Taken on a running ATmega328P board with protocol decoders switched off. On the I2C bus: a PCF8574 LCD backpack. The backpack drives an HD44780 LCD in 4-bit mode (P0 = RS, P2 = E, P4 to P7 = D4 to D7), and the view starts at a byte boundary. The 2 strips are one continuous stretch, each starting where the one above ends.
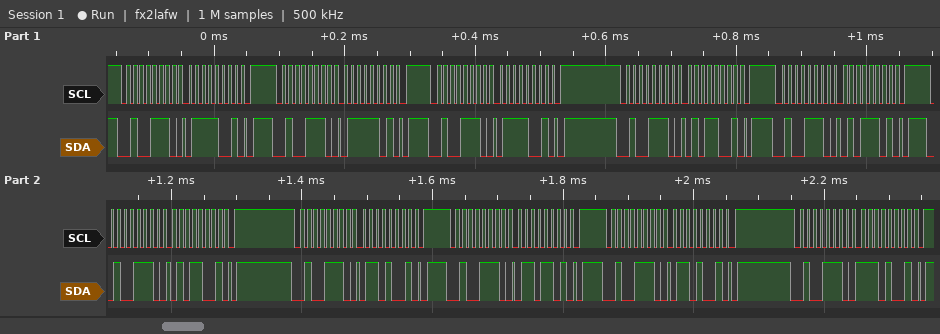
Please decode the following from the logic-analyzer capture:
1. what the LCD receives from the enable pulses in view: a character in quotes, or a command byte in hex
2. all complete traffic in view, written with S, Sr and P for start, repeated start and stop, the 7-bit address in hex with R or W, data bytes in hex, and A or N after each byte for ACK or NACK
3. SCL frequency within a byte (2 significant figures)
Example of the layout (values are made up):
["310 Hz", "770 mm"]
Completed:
["'u'", "S 27W A 79 A P S 27W A 7D A P S 27W A 79 A P S 27W A 59 A P S 27W A 5D A P S 27W A 59 A P S 27W A 69 A P S 27W A 6D A P S 27W A 69 A P S 27W A E9 A P", "100 kHz"]
